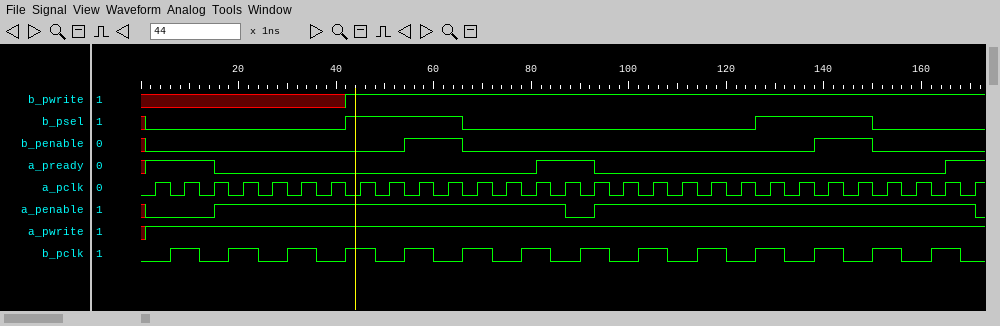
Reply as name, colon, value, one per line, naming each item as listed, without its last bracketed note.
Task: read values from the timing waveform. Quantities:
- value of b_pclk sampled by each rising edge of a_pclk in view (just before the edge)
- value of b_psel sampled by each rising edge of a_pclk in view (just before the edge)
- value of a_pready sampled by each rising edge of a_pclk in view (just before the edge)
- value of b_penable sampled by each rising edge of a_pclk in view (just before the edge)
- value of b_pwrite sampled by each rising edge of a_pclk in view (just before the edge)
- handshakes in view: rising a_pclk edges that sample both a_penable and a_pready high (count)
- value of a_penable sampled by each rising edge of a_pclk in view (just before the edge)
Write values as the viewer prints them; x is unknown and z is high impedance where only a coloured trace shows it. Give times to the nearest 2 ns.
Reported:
value of b_pclk sampled by each rising edge of a_pclk in view: 0 1 0 1 0 1 0 1 0 1 0 1 0 1 0 1 0 1 0 1 0 1 0 1 0 1 0 1 0
value of b_psel sampled by each rising edge of a_pclk in view: 0 0 0 0 0 0 0 1 1 1 1 0 0 0 0 0 0 0 0 0 0 1 1 1 1 0 0 0 0
value of a_pready sampled by each rising edge of a_pclk in view: 1 1 1 0 0 0 0 0 0 0 0 0 0 0 1 1 0 0 0 0 0 0 0 0 0 0 0 0 1
value of b_penable sampled by each rising edge of a_pclk in view: 0 0 0 0 0 0 0 0 0 1 1 0 0 0 0 0 0 0 0 0 0 0 0 1 1 0 0 0 0
value of b_pwrite sampled by each rising edge of a_pclk in view: x x x x x x x 1 1 1 1 1 1 1 1 1 1 1 1 1 1 1 1 1 1 1 1 1 1
handshakes in view: rising a_pclk edges that sample both a_penable and a_pready high: 2
value of a_penable sampled by each rising edge of a_pclk in view: 0 0 0 1 1 1 1 1 1 1 1 1 1 1 1 0 1 1 1 1 1 1 1 1 1 1 1 1 1
